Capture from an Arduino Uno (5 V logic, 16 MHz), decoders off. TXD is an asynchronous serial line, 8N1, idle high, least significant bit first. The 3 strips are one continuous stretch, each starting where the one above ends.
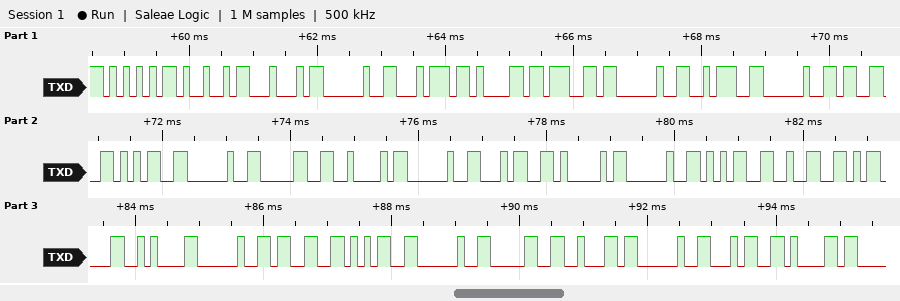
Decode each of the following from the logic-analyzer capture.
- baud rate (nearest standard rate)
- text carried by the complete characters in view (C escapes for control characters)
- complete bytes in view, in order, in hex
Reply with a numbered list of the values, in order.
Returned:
1. 9600 baud
2. "UID tag : 35 0B 4A 52\r\n 35 0b 4a"
3. 55 49 44 20 74 61 67 20 3A 20 33 35 20 30 42 20 34 41 20 35 32 0D 0A 20 33 35 20 30 62 20 34 61
